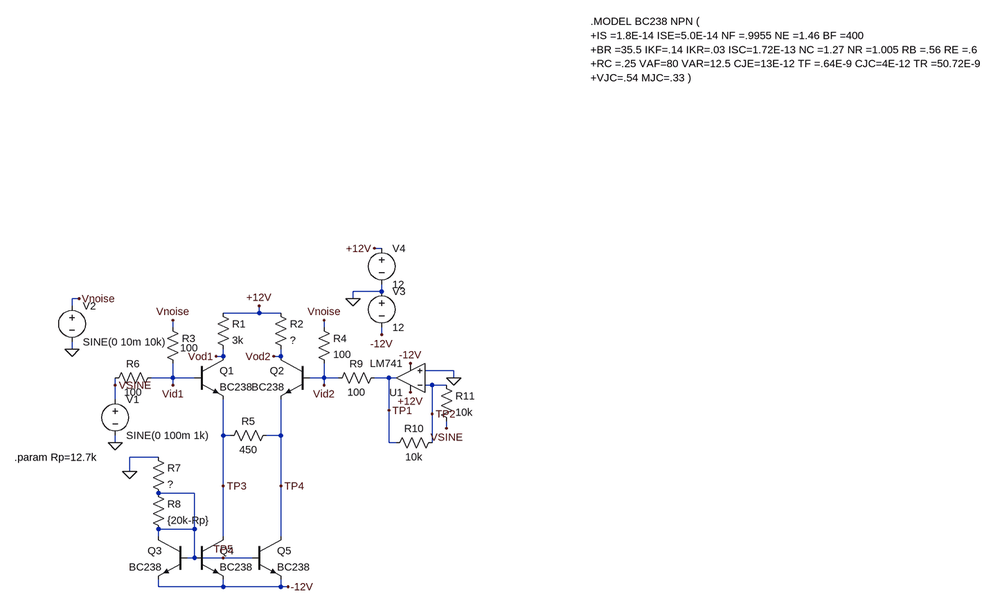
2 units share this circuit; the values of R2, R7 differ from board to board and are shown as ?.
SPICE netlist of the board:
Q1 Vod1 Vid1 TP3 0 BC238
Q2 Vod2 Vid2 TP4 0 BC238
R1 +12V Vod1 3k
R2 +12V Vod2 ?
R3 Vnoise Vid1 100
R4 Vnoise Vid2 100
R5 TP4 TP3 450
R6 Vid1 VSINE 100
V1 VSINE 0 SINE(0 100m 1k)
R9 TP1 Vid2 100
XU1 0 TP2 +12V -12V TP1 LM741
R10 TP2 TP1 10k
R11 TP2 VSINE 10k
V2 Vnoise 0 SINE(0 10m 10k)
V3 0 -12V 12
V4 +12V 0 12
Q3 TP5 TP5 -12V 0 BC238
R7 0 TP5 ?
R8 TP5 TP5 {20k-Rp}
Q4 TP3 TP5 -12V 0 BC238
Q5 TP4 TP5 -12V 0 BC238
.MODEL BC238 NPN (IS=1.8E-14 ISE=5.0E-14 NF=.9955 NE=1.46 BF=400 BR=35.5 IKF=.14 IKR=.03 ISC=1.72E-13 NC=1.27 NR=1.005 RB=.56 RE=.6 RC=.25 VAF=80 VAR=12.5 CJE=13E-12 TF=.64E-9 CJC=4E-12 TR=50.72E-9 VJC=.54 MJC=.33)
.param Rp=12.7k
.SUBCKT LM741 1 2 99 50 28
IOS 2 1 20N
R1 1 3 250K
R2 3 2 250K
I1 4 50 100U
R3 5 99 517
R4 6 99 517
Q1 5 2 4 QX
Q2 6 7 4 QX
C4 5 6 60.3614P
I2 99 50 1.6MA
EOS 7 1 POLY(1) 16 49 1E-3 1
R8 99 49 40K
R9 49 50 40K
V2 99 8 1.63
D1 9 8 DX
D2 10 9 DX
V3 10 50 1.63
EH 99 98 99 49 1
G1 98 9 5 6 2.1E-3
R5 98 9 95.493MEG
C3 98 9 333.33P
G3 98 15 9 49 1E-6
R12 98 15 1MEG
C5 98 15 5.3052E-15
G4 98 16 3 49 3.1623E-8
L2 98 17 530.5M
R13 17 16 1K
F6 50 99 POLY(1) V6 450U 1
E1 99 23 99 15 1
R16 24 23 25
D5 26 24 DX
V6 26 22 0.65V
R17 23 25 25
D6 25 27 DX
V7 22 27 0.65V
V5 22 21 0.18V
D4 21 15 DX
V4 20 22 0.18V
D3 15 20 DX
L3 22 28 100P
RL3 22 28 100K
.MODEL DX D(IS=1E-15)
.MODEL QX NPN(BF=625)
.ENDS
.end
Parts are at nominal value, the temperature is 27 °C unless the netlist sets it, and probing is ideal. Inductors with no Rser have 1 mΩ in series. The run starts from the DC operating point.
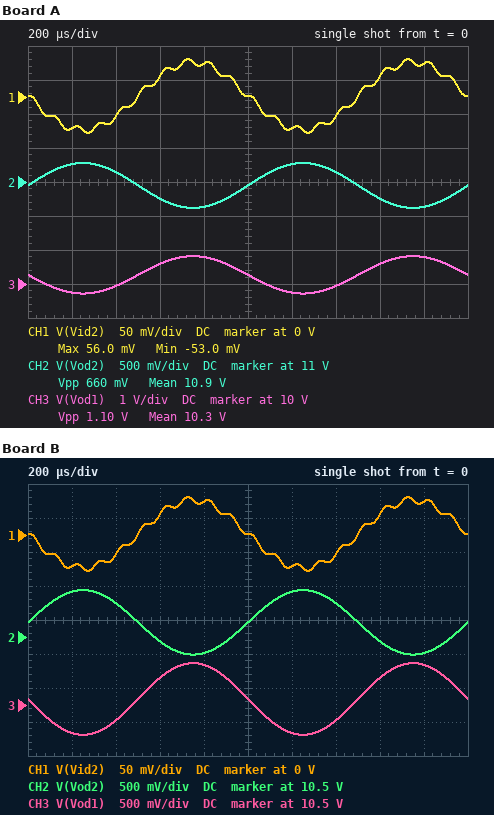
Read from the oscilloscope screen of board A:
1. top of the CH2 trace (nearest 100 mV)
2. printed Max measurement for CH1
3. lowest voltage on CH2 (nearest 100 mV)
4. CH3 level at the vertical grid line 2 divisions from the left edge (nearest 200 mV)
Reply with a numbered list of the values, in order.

1. 11.3 V
2. 56.0 mV
3. 10.6 V
4. 10.0 V
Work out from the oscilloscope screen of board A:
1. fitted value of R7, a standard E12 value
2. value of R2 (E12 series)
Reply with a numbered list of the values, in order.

1. 22 kΩ
2. 1.8 kΩ
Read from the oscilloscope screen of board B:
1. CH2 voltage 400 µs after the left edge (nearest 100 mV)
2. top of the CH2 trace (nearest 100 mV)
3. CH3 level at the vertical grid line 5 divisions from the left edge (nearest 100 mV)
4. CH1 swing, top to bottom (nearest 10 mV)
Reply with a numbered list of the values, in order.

1. 11.0 V
2. 11.2 V
3. 10.6 V
4. 110 mV
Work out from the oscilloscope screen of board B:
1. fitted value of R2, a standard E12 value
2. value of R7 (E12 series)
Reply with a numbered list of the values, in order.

1. 2.7 kΩ
2. 27 kΩ
